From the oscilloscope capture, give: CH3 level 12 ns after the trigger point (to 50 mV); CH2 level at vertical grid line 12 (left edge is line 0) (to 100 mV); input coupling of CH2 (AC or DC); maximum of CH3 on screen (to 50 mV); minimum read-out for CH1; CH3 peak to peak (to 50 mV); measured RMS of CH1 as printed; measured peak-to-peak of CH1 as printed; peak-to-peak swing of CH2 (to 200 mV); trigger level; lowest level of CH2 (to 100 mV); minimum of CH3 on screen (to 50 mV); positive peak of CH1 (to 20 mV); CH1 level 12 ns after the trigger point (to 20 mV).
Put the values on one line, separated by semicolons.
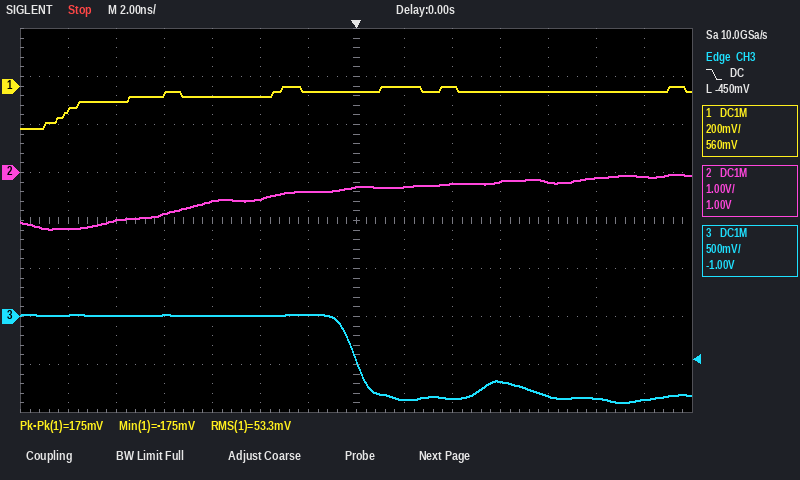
-850 mV; -100 mV; DC; 0 mV; -175 mV; 900 mV; 53.3 mV; 175 mV; 1.2 V; -450 mV; -1.2 V; -900 mV; 0 mV; -20 mV
